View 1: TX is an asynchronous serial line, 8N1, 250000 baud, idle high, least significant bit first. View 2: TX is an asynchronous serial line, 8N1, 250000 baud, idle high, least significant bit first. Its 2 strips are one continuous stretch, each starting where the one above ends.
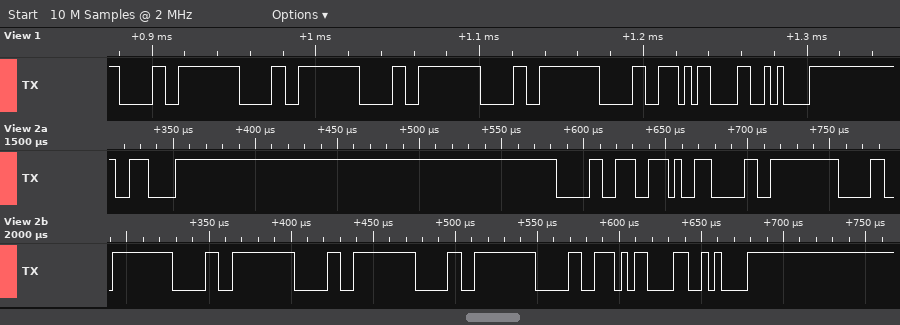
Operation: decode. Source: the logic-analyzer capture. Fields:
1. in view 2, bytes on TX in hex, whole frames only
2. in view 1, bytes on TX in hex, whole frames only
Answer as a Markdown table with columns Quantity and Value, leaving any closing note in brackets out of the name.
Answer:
| Quantity | Value |
|---|---|
| in view 2, bytes on TX in hex, whole frames only | 0x0E 0x30 0x2E 0x30 0x30 0x30 0x30 0x30 0x30 0x0D 0x0A |
| in view 1, bytes on TX in hex, whole frames only | 0x30 0x30 0x30 0x30 0x30 0x0D 0x0A |
